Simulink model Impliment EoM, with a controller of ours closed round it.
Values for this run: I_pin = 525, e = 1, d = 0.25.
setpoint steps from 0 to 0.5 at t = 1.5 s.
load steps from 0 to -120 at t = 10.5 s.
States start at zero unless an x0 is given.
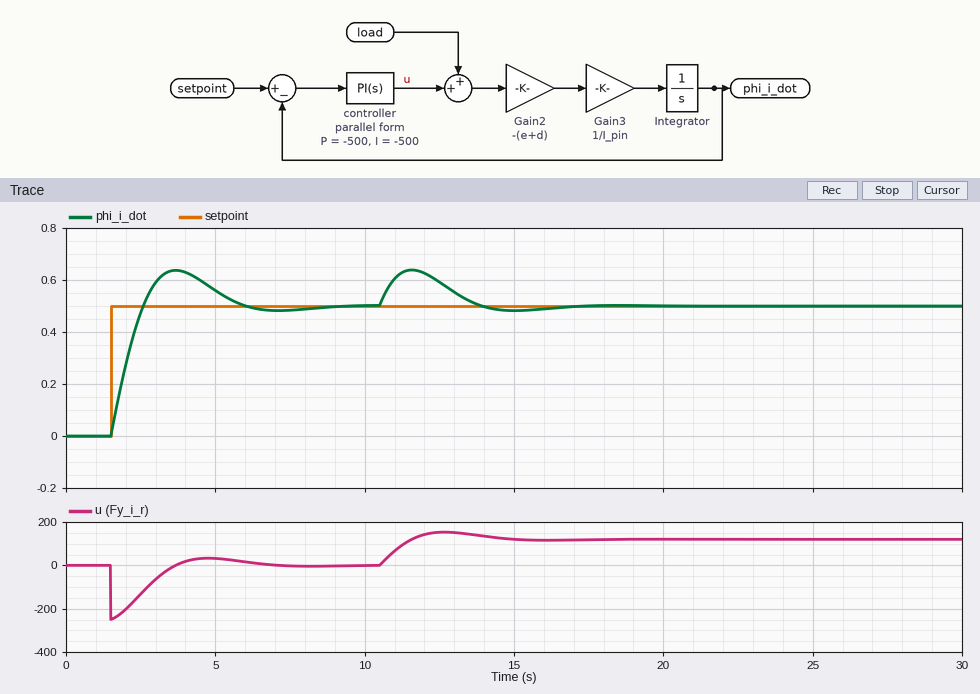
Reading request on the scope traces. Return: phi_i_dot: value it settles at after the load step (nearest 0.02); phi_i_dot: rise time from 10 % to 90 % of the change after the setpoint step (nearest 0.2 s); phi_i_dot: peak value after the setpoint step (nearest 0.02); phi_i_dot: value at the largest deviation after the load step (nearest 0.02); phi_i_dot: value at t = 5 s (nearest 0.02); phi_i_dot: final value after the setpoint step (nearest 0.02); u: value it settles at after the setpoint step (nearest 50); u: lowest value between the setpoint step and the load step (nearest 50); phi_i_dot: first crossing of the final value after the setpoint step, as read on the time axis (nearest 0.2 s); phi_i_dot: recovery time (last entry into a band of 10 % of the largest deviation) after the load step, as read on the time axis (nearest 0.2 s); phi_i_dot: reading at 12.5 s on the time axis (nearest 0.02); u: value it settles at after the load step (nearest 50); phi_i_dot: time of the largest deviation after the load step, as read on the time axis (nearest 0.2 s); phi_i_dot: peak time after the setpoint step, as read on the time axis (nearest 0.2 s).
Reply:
0.50
0.8 s
0.64
0.64
0.56
0.50
0
-250
2.6 s
15.8 s
0.60
100
11.6 s
3.6 s
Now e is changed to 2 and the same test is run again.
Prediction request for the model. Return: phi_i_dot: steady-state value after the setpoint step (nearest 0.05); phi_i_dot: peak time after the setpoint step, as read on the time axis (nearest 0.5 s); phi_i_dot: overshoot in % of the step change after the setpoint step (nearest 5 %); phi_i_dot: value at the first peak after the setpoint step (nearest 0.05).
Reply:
0.50
3.0 s
20 %
0.60
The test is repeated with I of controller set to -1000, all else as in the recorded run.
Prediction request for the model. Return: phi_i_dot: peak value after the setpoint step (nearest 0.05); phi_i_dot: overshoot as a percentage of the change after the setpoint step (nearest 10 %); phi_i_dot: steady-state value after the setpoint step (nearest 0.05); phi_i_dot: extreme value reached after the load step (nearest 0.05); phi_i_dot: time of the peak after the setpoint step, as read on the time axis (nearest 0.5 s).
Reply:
0.70
40 %
0.50
0.60
3.0 s
